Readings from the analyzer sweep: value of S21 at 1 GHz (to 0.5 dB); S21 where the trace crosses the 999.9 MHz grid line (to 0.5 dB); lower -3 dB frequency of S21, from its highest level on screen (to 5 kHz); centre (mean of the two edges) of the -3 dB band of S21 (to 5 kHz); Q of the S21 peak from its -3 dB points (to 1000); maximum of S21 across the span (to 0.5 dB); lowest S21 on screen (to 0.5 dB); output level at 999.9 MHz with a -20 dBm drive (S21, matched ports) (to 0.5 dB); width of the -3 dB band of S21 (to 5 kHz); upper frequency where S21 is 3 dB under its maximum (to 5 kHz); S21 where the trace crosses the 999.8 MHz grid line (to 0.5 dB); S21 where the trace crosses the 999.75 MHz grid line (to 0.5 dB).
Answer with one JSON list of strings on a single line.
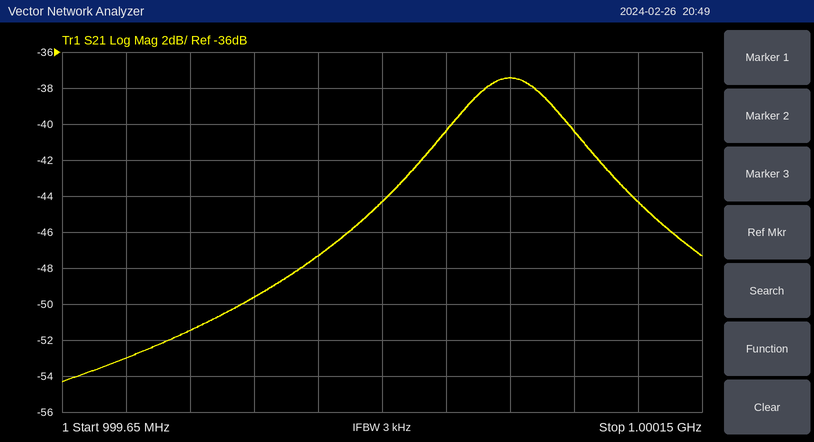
["-37.5 dB", "-44.5 dB", "999.950 MHz", "1.000000 GHz", "10000", "-37.5 dB", "-54.5 dB", "-64.5 dBm", "100 kHz", "1.000050 GHz", "-49.5 dB", "-51.5 dB"]
